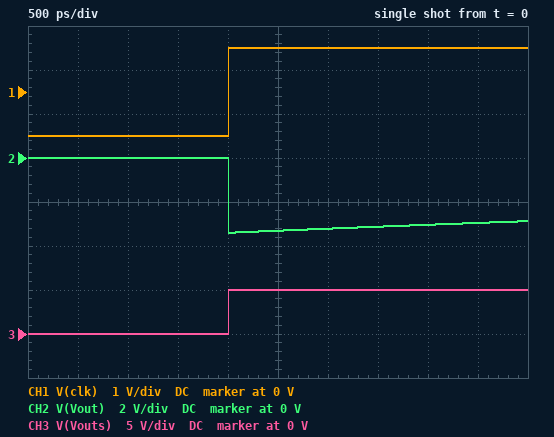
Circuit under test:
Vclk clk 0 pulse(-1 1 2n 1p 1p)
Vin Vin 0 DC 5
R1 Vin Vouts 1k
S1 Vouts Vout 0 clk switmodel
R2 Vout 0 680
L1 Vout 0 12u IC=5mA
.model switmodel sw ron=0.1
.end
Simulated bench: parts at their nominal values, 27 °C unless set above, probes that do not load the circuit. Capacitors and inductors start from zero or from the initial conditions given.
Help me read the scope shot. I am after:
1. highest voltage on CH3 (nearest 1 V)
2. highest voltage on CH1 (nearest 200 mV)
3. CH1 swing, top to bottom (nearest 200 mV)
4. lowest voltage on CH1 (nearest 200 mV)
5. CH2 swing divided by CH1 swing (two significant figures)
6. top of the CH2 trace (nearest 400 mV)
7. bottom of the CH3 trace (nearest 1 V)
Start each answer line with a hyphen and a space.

- 5 V
- 1.0 V
- 2.0 V
- -1.0 V
- 1.7
- 0 V
- 0 V
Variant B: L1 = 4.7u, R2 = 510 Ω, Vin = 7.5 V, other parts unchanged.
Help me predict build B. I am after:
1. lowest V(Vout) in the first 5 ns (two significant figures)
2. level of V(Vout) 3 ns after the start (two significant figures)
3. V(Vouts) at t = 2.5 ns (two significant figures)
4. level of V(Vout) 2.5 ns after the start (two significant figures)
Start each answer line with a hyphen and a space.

- -2.7 V
- -2.4 V
- 7.5 V
- -2.6 V
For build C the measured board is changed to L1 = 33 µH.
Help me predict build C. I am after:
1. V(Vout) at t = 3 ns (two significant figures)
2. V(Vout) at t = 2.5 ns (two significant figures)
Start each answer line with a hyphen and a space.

- -3.3 V
- -3.4 V
